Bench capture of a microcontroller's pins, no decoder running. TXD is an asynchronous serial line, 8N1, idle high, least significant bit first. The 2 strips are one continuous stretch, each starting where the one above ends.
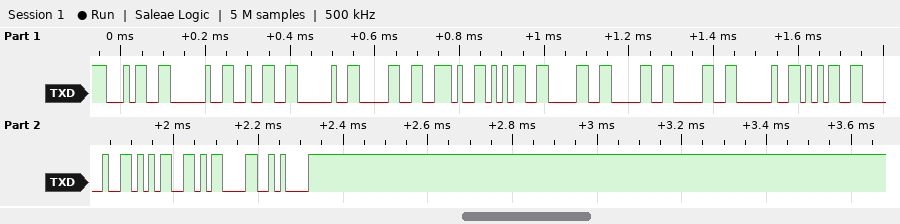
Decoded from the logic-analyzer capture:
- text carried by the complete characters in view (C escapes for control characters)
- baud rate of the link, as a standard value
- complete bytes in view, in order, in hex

"4 2 0.5000 5 5\r\n"
74880 baud
0x34 0x20 0x32 0x20 0x30 0x2E 0x35 0x30 0x30 0x30 0x20 0x35 0x20 0x35 0x0D 0x0A
